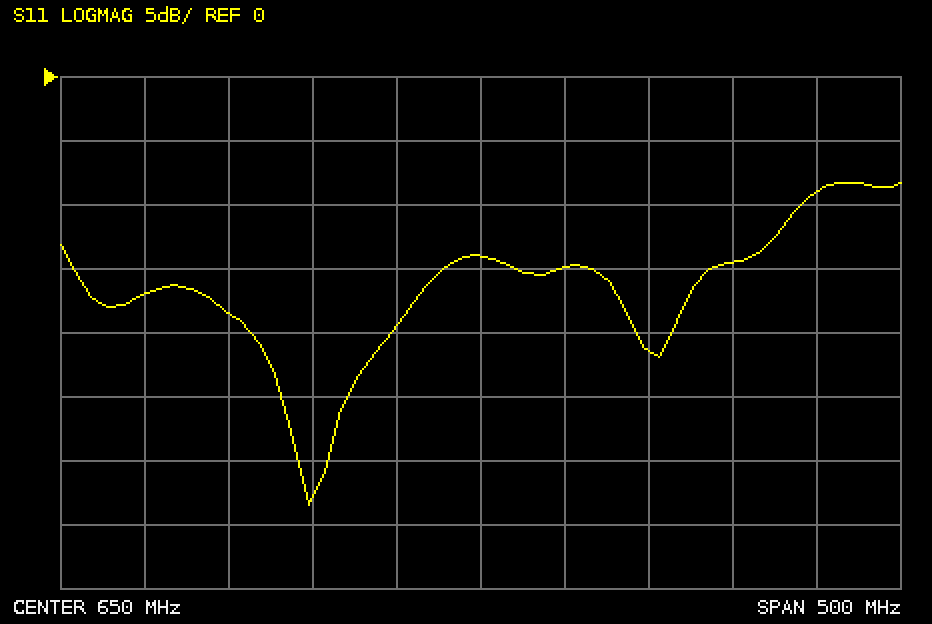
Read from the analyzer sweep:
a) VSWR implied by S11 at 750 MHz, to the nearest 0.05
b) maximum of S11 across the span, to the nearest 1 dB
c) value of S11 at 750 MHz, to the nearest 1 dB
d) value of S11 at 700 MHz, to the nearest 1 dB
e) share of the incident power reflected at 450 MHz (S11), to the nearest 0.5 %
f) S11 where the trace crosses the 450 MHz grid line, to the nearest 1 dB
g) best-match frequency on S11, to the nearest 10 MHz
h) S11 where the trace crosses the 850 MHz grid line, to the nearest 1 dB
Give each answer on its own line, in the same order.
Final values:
1.20
-8 dB
-21 dB
-15 dB
2.0 %
-17 dB
550 MHz
-9 dB
